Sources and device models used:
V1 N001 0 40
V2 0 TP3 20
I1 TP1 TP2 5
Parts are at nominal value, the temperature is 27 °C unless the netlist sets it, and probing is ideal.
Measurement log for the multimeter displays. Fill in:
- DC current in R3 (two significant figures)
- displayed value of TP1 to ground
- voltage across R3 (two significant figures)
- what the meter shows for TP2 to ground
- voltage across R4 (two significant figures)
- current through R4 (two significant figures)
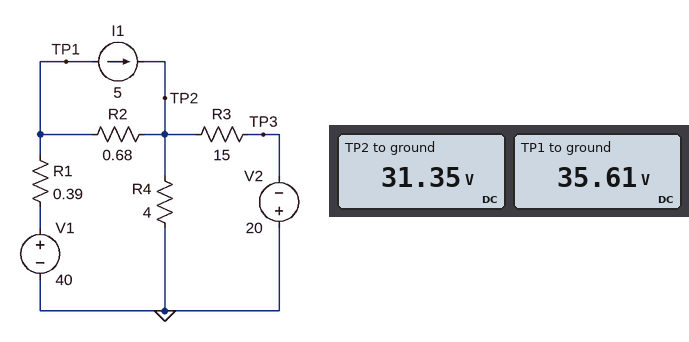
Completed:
3.4 A
35.61 V
51 V
31.35 V
31 V
7.8 A
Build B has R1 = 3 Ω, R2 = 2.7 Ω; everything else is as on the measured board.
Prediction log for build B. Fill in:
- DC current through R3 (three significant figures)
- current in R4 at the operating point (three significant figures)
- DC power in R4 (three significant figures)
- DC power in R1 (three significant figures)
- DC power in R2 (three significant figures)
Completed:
2.42 A
4.09 A
66.9 W
127 W
6.20 W
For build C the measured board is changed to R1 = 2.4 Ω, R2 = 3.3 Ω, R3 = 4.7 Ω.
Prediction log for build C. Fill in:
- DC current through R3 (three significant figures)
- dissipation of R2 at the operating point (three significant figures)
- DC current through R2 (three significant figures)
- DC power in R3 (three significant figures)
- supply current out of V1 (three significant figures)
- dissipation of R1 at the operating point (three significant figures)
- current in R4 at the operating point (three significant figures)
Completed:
6.14 A
37.2 W
3.36 A
177 W
8.36 A
168 W
2.22 A
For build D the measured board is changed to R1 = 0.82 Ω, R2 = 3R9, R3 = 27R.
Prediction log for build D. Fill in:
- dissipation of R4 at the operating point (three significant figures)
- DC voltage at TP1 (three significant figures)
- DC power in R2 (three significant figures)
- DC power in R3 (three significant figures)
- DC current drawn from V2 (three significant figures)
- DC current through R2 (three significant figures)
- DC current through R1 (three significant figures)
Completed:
141 W
33.8 V
25.7 W
71.0 W
1.62 A
2.57 A
7.57 A
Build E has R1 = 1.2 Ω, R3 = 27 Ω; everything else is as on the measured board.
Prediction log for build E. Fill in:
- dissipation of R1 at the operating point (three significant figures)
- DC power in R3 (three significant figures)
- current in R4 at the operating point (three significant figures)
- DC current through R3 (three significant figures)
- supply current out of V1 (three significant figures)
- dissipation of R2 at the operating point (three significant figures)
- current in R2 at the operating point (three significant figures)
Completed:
88.2 W
82.8 W
6.82 A
1.75 A
8.57 A
8.68 W
3.57 A
